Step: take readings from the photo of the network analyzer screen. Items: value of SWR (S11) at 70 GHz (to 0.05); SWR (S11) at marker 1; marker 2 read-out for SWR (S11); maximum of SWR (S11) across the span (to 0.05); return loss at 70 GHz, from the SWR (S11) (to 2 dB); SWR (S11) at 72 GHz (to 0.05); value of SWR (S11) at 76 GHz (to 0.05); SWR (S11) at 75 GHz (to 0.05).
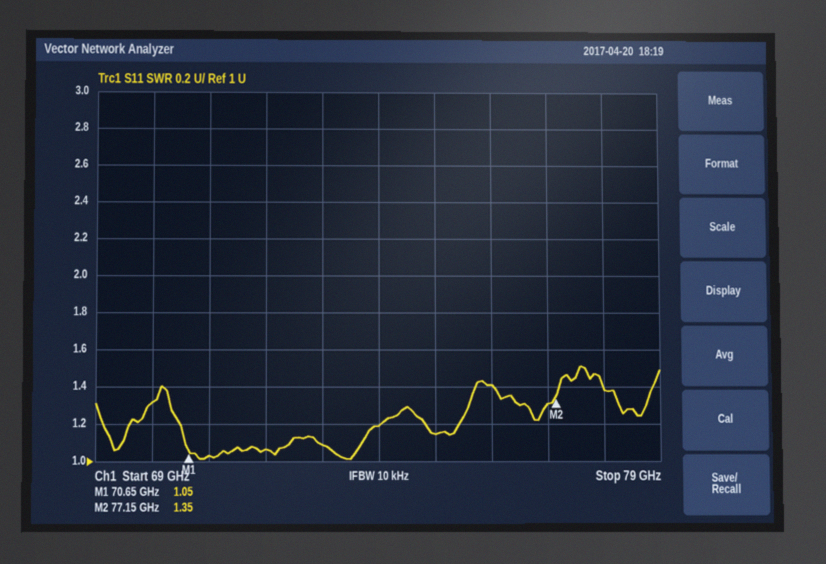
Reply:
1.30
1.05
1.35
1.50
18 dB
1.05
1.40
1.15
